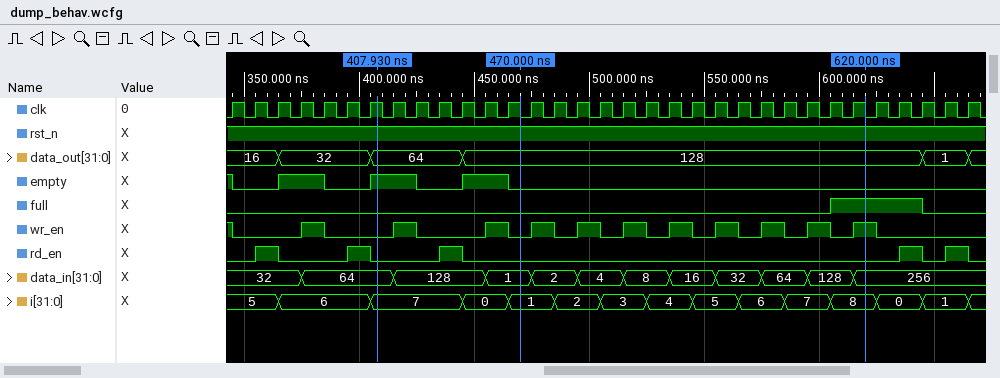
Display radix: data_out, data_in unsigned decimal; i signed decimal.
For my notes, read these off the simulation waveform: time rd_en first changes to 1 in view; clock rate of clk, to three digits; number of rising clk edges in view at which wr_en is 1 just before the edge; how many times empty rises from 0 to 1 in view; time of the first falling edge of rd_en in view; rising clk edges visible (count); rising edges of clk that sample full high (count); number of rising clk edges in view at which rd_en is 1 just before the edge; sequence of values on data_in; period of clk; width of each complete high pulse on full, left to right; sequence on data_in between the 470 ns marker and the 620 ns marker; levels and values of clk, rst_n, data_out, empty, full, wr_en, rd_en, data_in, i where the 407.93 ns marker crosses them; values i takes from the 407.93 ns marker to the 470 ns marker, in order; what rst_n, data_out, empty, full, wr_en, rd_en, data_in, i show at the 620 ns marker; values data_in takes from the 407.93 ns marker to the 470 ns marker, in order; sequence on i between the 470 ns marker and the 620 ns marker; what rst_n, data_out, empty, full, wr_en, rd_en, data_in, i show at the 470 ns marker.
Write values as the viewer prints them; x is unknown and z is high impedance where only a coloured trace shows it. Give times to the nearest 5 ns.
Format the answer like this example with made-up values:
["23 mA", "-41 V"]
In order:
["355 ns", "100 MHz", "12", "3", "365 ns", "33", "4", "5", "32, 64, 128, 1, 2, 4, 8, 16, 32, 64, 128, 256", "10 ns", "40 ns", "1, 2, 4, 8, 16, 32, 64, 128, 256", "clk=1, rst_n=1, data_out=64, empty=1, full=0, wr_en=0, rd_en=0, data_in=64, i=7", "7, 0, 1", "rst_n=1, data_out=128, empty=0, full=1, wr_en=1, rd_en=0, data_in=256, i=8", "64, 128, 1", "1, 2, 3, 4, 5, 6, 7, 8", "rst_n=1, data_out=128, empty=0, full=0, wr_en=0, rd_en=0, data_in=1, i=1"]
